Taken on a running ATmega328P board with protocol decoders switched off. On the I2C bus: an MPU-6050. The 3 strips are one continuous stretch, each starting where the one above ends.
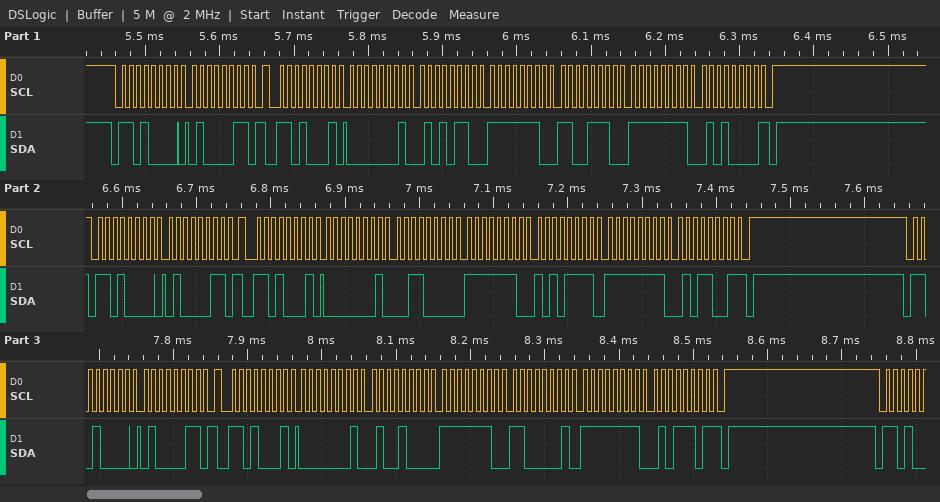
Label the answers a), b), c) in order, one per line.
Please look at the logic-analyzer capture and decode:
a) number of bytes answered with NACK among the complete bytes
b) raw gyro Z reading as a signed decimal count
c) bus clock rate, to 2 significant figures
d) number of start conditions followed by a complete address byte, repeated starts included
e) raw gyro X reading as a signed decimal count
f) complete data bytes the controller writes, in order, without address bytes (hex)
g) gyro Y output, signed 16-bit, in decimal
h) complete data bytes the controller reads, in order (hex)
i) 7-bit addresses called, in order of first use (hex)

a) 3
b) -176
c) 100 kHz
d) 6
e) 342
f) 43 43 43
g) -306
h) 01 56 FE CE FF 50 01 30 FE AF FF 59 01 48 FE C1 FF 5D
i) 0x68
